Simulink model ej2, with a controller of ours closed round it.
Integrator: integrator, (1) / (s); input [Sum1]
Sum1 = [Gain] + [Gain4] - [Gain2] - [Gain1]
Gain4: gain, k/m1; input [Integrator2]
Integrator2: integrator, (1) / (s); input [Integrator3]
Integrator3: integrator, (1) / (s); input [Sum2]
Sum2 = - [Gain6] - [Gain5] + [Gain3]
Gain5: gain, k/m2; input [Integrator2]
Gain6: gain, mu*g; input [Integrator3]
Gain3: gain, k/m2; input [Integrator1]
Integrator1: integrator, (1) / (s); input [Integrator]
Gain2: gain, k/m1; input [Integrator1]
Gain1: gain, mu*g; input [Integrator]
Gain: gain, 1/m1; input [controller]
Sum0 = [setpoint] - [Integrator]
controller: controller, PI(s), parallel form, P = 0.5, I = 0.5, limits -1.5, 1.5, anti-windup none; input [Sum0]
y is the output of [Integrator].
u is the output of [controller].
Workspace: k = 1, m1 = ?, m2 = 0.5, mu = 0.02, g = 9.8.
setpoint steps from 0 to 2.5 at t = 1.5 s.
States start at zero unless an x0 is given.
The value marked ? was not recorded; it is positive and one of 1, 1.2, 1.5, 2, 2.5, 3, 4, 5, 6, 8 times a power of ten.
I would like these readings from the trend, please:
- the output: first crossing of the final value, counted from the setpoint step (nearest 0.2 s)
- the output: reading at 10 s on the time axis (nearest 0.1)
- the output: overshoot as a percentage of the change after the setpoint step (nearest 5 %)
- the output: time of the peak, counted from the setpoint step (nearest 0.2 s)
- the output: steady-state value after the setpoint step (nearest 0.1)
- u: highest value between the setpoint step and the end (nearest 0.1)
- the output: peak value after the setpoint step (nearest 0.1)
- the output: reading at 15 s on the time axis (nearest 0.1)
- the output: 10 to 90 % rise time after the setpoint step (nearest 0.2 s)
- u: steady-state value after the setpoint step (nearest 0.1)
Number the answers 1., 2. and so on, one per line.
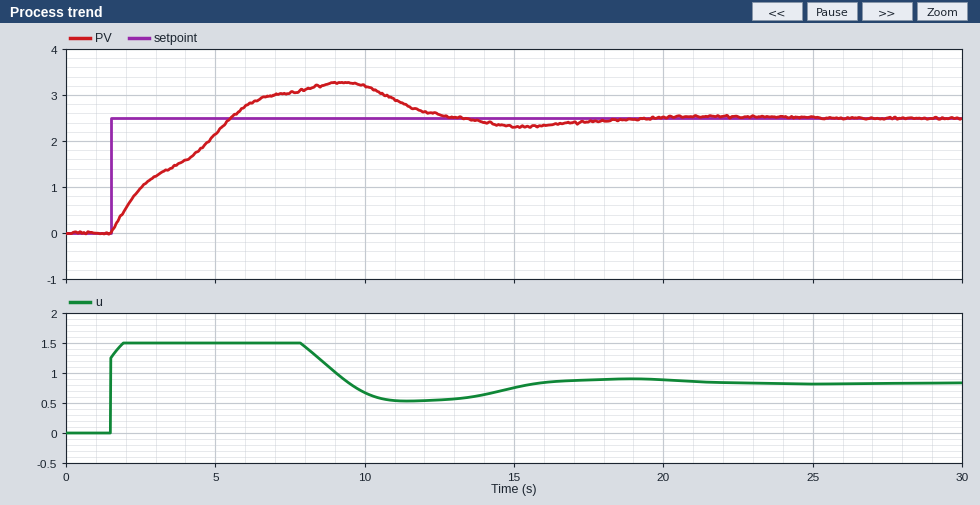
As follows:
1. 4.0 s
2. 3.2
3. 30 %
4. 7.8 s
5. 2.5
6. 1.5
7. 3.3
8. 2.3
9. 3.4 s
10. 0.8
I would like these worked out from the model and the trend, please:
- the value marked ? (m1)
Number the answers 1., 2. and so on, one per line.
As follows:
1. 1.2
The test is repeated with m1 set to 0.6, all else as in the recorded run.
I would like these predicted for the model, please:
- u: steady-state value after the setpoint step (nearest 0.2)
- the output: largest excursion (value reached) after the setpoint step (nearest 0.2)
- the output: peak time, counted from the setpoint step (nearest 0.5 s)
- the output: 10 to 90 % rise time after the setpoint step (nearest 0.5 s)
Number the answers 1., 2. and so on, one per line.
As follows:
1. 0.6
2. 3.2
3. 4.0 s
4. 2.5 s
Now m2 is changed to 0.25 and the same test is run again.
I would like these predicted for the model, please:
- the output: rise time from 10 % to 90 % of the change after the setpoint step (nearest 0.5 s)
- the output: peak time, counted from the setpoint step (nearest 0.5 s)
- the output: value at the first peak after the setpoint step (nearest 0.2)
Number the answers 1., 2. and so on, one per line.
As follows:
1. 2.5 s
2. 6.0 s
3. 3.2
